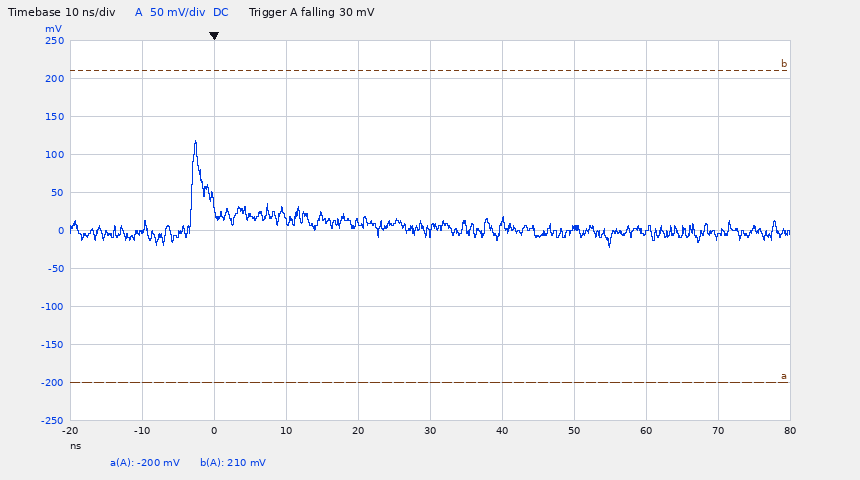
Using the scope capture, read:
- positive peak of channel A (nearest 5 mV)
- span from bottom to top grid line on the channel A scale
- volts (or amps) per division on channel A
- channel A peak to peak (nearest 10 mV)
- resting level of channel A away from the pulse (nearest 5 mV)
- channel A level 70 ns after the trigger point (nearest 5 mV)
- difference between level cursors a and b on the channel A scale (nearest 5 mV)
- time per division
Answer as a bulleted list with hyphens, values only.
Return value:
- 120 mV
- 500 mV
- 50 mV
- 140 mV
- 0 mV
- -10 mV
- 410 mV
- 10 ns
